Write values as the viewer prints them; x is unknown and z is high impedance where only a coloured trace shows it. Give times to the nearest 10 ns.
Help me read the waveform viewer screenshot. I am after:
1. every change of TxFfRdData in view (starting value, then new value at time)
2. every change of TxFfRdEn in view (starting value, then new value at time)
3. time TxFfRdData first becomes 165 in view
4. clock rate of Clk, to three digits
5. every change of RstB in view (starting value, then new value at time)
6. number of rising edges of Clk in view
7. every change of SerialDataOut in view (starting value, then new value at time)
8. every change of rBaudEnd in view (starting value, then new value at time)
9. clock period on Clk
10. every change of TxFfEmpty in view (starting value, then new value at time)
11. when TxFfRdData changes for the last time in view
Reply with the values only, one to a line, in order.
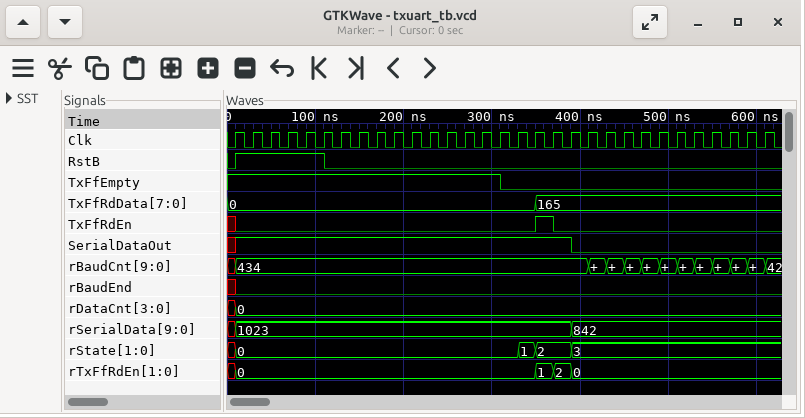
0, 165 at 350 ns
x, 0 at 10 ns, 1 at 350 ns, 0 at 370 ns
350 ns
50.0 MHz
0, 1 at 10 ns, 0 at 110 ns
31
x, 1 at 10 ns, 0 at 390 ns
x, 0 at 10 ns
20 ns
1, 0 at 310 ns
350 ns
